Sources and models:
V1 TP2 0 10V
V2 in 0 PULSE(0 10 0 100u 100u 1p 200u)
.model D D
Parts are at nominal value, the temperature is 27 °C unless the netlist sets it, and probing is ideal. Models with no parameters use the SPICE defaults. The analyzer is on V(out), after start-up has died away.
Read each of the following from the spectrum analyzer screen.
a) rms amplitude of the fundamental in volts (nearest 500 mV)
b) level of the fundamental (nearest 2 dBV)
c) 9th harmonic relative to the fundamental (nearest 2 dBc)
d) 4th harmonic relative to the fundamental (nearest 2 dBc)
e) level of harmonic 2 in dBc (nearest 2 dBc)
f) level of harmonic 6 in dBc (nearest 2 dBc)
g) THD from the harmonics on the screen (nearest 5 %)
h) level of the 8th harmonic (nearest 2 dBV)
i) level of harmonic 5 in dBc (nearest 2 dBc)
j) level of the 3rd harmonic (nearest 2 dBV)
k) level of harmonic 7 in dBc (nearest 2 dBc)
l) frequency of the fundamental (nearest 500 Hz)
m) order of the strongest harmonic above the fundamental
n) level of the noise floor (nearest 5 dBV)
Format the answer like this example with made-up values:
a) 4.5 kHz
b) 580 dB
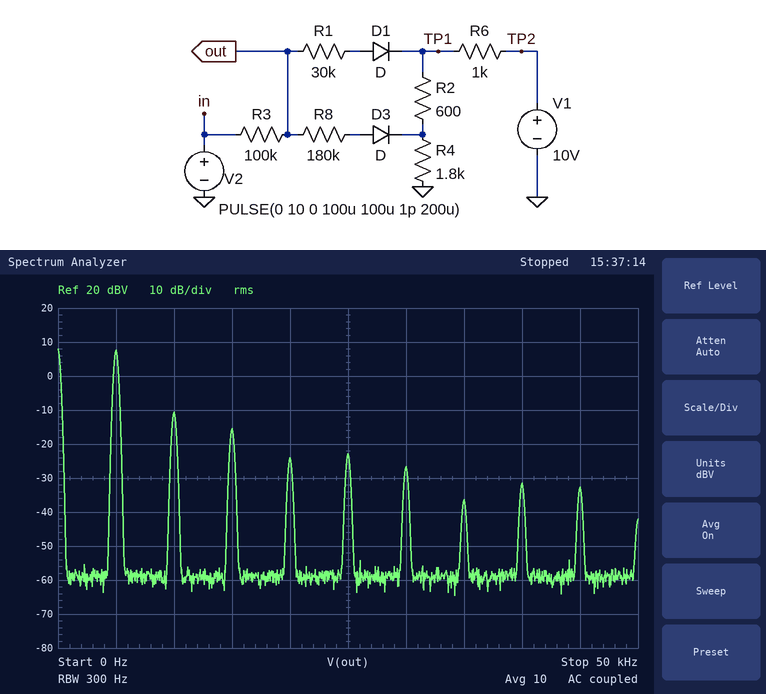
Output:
a) 2.5 V
b) 8 dBV
c) -40 dBc
d) -32 dBc
e) -18 dBc
f) -34 dBc
g) 15 %
h) -32 dBV
i) -30 dBc
j) -16 dBV
k) -44 dBc
l) 5.0 kHz
m) 2
n) -60 dBV
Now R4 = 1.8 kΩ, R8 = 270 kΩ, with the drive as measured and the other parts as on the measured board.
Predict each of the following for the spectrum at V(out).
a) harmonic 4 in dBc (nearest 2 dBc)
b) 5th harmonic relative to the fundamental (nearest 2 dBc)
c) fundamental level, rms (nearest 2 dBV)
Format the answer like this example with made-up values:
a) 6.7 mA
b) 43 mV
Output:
a) -30 dBc
b) -32 dBc
c) 8 dBV
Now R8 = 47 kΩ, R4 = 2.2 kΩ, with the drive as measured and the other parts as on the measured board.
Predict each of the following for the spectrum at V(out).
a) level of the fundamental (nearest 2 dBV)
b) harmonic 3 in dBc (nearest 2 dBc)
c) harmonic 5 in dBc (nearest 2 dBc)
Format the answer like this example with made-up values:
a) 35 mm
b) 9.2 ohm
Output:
a) 8 dBV
b) -26 dBc
c) -26 dBc
